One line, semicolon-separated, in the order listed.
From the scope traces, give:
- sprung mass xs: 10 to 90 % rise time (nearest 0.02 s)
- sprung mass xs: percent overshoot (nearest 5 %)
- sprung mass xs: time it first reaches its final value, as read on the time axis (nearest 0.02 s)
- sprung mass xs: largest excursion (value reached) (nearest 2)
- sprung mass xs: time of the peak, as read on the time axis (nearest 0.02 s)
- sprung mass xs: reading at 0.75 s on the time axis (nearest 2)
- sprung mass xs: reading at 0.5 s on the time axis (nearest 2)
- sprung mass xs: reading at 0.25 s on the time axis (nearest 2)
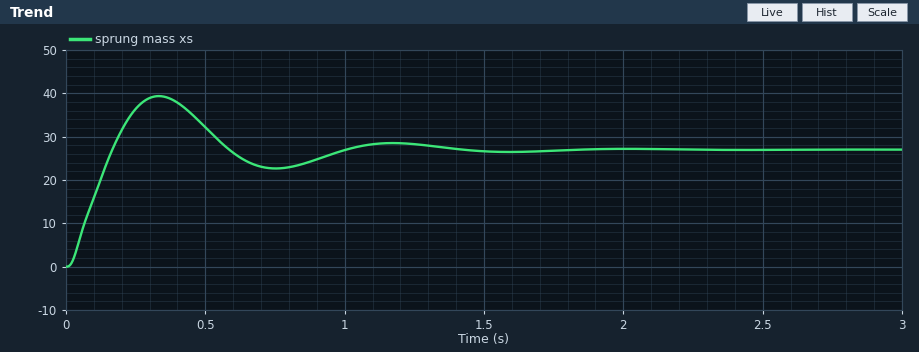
0.12 s; 45 %; 0.16 s; 40; 0.34 s; 22; 32; 36
